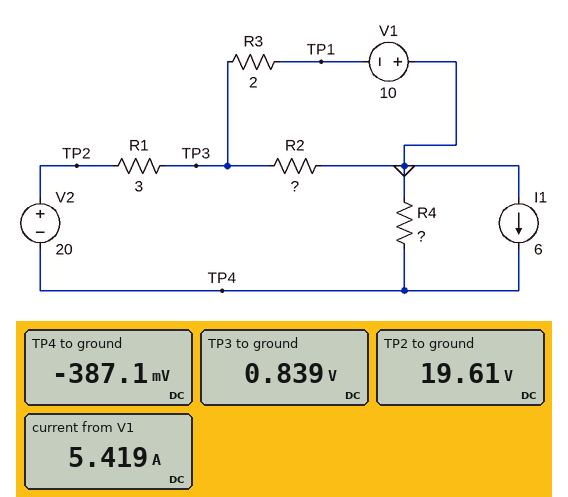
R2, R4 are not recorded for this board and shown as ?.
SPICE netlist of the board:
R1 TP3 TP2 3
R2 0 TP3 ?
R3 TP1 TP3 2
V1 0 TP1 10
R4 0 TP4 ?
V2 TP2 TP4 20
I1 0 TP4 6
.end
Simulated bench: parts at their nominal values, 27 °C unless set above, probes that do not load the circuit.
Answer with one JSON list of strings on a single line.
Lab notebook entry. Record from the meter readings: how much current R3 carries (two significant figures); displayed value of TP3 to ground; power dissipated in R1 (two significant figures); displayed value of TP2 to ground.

["5.4 A", "0.839 V", "120 W", "19.61 V"]
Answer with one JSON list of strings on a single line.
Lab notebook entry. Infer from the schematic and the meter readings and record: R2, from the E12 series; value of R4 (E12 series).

["1 Ω", "1.5 Ω"]
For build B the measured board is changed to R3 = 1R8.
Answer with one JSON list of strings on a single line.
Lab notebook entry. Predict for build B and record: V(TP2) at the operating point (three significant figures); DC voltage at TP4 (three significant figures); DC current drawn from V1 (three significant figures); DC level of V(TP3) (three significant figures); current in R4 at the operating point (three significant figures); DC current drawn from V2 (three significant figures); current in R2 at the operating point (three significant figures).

["19.5 V", "-500 mV", "5.83 A", "500 mV", "333 mA", "6.33 A", "500 mA"]
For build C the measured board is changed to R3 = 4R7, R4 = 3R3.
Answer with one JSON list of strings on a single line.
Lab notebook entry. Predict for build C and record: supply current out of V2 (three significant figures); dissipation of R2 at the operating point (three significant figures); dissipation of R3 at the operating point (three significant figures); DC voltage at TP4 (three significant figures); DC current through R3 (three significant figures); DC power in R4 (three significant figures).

["5.83 A", "9.33 W", "36.3 W", "553 mV", "2.78 A", "92.5 mW"]
